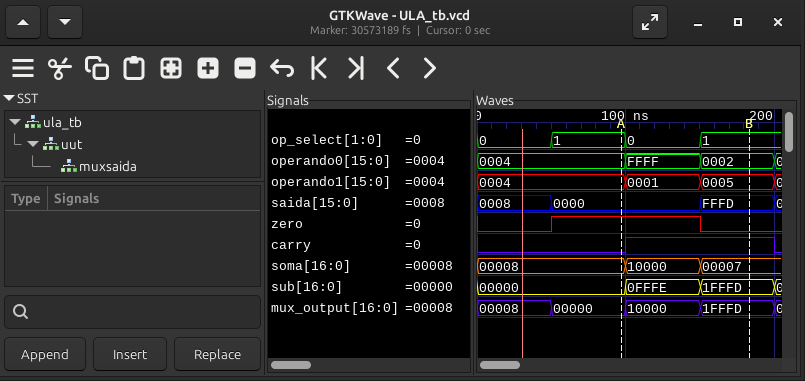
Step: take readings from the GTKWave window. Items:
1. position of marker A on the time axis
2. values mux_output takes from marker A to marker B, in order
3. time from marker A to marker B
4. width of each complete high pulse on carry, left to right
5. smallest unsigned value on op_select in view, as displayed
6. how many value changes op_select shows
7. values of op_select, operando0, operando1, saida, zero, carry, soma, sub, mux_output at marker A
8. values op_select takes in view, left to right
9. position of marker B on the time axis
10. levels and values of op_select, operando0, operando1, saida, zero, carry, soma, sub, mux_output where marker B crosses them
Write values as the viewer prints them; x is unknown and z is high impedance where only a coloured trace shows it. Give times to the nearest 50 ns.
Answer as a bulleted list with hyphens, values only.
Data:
- 100 ns
- 00000, 10000, 1FFFD
- 100 ns
- 100 ns
- 0
- 3
- op_select=1, operando0=0004, operando1=0004, saida=0000, zero=1, carry=0, soma=00008, sub=00000, mux_output=00000
- 0, 1, 0, 1
- 200 ns
- op_select=1, operando0=0002, operando1=0005, saida=FFFD, zero=0, carry=1, soma=00007, sub=1FFFD, mux_output=1FFFD
